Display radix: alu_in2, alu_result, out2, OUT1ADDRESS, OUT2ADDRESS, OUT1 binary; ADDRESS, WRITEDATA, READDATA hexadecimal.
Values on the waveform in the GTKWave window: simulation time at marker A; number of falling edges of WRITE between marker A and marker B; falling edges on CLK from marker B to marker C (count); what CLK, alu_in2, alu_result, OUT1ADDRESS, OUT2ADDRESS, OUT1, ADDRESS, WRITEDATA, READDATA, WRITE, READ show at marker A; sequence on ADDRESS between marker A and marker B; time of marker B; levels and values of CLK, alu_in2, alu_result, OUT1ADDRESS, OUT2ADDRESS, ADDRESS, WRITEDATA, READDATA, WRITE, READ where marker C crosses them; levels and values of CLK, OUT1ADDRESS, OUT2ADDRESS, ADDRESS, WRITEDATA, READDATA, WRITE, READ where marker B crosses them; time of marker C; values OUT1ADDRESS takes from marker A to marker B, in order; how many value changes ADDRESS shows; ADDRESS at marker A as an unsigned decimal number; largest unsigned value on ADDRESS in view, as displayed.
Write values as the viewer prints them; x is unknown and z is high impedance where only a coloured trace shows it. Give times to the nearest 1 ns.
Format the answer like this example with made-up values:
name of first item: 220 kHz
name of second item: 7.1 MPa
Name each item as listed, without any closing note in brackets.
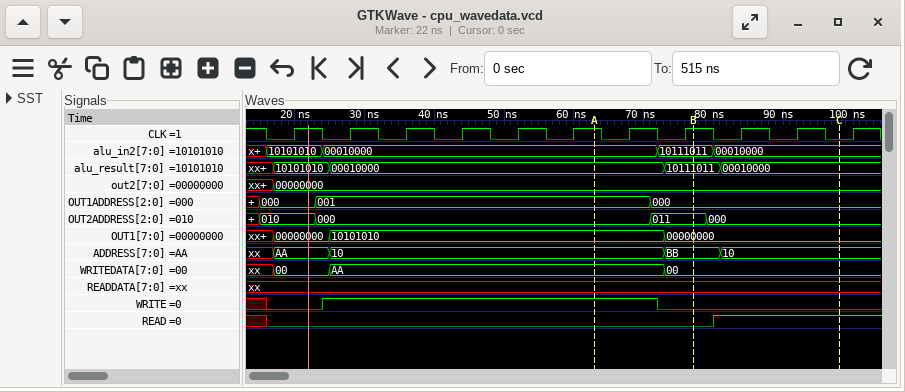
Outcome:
simulation time at marker A: 63 ns
number of falling edges of WRITE between marker A and marker B: 1
falling edges on CLK from marker B to marker C: 3
what CLK, alu_in2, alu_result, OUT1ADDRESS, OUT2ADDRESS, OUT1, ADDRESS, WRITEDATA, READDATA, WRITE, READ show at marker A: CLK=1, alu_in2=00010000, alu_result=00010000, OUT1ADDRESS=001, OUT2ADDRESS=000, OUT1=10101010, ADDRESS=10, WRITEDATA=AA, READDATA=xx, WRITE=1, READ=0
sequence on ADDRESS between marker A and marker B: 10, BB
time of marker B: 77 ns
levels and values of CLK, alu_in2, alu_result, OUT1ADDRESS, OUT2ADDRESS, ADDRESS, WRITEDATA, READDATA, WRITE, READ where marker C crosses them: CLK=0, alu_in2=00010000, alu_result=00010000, OUT1ADDRESS=000, OUT2ADDRESS=000, ADDRESS=10, WRITEDATA=00, READDATA=xx, WRITE=0, READ=1
levels and values of CLK, OUT1ADDRESS, OUT2ADDRESS, ADDRESS, WRITEDATA, READDATA, WRITE, READ where marker B crosses them: CLK=1, OUT1ADDRESS=000, OUT2ADDRESS=011, ADDRESS=BB, WRITEDATA=00, READDATA=xx, WRITE=0, READ=0
time of marker C: 98 ns
values OUT1ADDRESS takes from marker A to marker B, in order: 001, 000
how many value changes ADDRESS shows: 4
ADDRESS at marker A as an unsigned decimal number: 16
largest unsigned value on ADDRESS in view, as displayed: BB
